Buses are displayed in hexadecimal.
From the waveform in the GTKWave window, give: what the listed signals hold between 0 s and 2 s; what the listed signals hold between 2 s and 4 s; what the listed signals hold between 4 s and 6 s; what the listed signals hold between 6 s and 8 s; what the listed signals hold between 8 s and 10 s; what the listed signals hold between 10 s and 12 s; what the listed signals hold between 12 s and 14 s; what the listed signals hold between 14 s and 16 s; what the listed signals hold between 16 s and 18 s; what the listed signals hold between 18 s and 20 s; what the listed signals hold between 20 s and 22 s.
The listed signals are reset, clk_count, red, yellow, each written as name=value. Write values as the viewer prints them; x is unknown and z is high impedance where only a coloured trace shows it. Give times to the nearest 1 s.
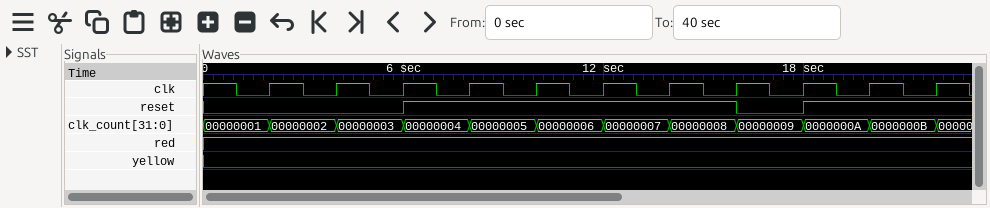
reset=0, clk_count=00000001, red=1, yellow=0
reset=0, clk_count=00000002, red=1, yellow=0
reset=0, clk_count=00000003, red=1, yellow=0
reset=1, clk_count=00000004, red=1, yellow=0
reset=1, clk_count=00000005, red=1, yellow=0
reset=1, clk_count=00000006, red=1, yellow=0
reset=1, clk_count=00000007, red=1, yellow=0
reset=1, clk_count=00000008, red=1, yellow=0
reset=0, clk_count=00000009, red=1, yellow=0
reset=1, clk_count=0000000A, red=1, yellow=0
reset=1, clk_count=0000000B, red=1, yellow=0
